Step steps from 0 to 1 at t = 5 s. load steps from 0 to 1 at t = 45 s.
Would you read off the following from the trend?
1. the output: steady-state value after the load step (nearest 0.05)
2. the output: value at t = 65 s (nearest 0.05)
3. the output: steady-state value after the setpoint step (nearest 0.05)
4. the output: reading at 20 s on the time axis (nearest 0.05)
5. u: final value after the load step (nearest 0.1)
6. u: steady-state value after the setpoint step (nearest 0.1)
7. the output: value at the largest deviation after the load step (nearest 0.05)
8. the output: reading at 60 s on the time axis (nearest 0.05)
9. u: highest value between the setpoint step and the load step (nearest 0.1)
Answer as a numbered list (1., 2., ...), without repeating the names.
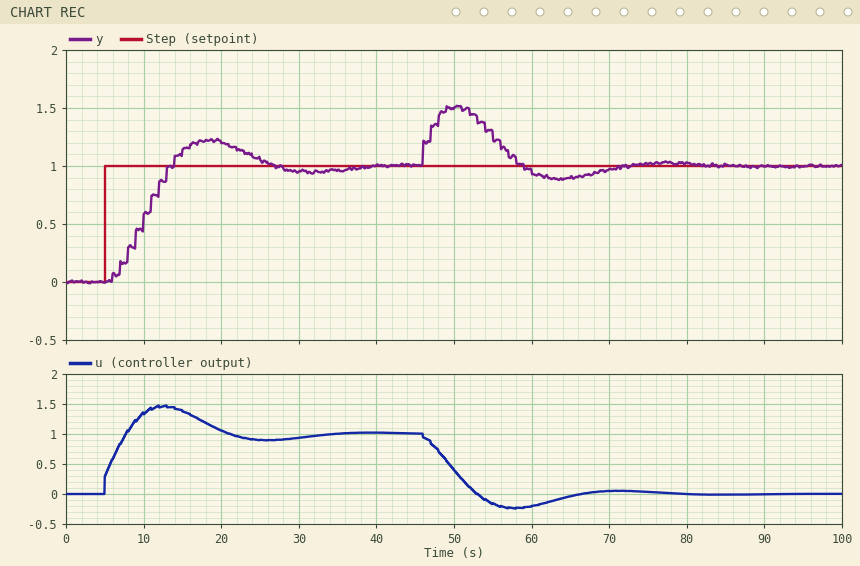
1. 1.00
2. 0.90
3. 1.00
4. 1.20
5. 0.0
6. 1.0
7. 1.50
8. 0.95
9. 1.5
